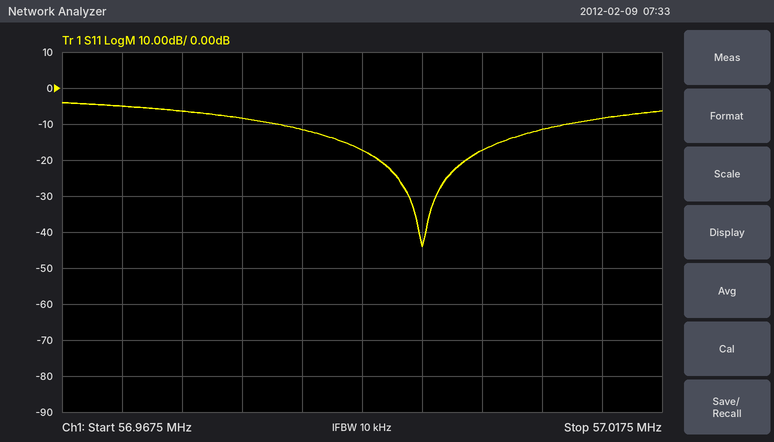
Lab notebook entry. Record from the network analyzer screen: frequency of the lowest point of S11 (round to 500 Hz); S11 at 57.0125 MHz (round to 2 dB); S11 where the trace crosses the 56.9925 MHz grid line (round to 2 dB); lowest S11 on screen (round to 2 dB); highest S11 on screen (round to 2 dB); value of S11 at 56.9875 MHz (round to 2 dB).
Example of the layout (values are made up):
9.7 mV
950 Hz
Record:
56.9975 MHz
-8 dB
-18 dB
-44 dB
-4 dB
-12 dB
